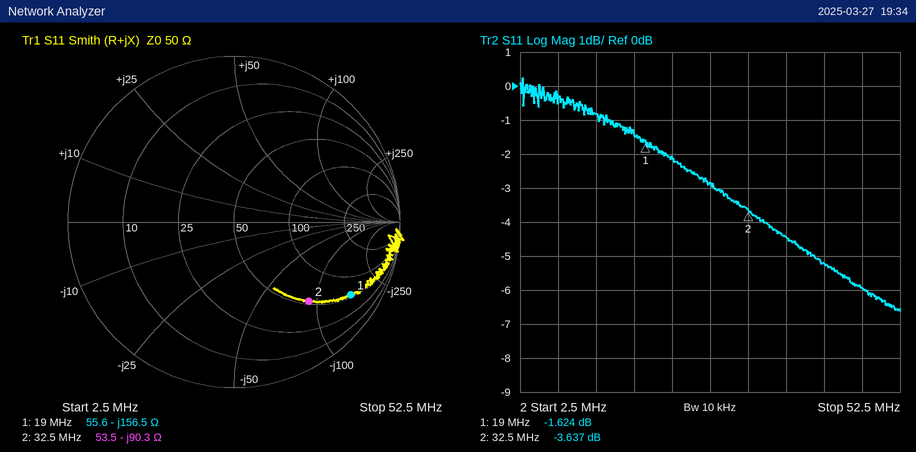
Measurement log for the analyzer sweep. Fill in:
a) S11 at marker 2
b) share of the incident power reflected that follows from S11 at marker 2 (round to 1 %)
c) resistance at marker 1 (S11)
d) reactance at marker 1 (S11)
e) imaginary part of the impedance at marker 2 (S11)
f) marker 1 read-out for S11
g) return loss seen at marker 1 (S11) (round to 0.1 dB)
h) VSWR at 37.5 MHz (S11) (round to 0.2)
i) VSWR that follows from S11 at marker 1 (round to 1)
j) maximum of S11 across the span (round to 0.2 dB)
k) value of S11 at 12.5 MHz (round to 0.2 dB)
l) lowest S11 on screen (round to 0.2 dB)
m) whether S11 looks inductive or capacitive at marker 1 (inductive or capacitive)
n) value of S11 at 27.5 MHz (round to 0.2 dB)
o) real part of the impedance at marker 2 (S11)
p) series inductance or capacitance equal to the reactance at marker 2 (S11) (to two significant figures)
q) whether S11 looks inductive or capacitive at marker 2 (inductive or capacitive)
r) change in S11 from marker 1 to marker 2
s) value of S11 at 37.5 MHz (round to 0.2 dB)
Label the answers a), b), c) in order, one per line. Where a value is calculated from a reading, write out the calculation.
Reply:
a) -3.637 dB
b) 10^(-3.637/10) ≈ 43 %
c) 55.6 Ω
d) -156.5 Ω
e) -90.3 Ω
f) -1.624 dB
g) 1.6 dB
h) |Γ| = 10^(-4.4/20) = 0.6026; VSWR = (1 + 0.6026)/(1 − 0.6026) ≈ 4.0
i) (1 + 0.8295)/(1 − 0.8295) ≈ 11
j) 0.2 dB
k) -0.8 dB
l) -6.6 dB
m) capacitive
n) -2.8 dB
o) 53.5 Ω
p) C = 1/(2π × 32.5 MHz × 90.3 Ω) ≈ 54 pF
q) capacitive
r) -3.637 − (-1.624) = -2.013 dB
s) -4.4 dB
